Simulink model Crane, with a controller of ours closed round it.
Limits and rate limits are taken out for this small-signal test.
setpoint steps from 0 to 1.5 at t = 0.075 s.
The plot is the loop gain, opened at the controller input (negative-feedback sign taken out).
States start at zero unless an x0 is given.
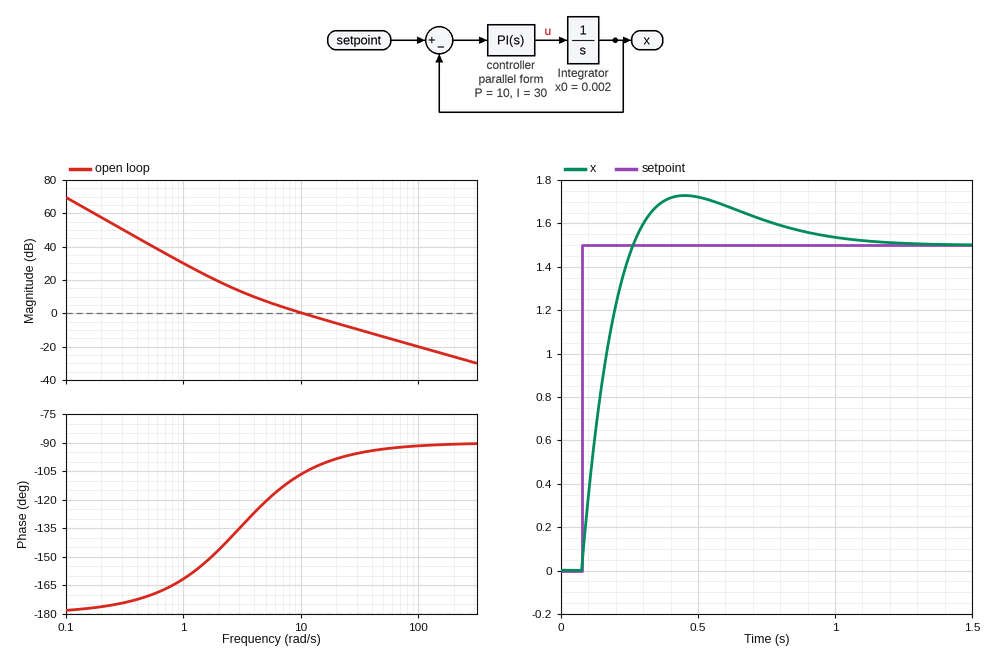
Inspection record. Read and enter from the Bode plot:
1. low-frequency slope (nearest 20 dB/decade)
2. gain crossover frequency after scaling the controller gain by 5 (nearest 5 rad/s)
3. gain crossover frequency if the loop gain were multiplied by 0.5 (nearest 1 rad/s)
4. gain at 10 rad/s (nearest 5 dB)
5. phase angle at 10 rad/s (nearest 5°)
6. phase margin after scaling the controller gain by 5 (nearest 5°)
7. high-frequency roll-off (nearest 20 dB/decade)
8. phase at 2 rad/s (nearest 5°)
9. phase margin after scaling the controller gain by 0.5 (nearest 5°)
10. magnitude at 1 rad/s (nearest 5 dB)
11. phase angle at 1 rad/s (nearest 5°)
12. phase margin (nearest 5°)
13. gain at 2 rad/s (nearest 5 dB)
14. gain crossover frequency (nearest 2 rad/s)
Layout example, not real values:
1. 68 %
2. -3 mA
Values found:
1. -40 dB/decade
2. 50 rad/s
3. 6 rad/s
4. 0 dB
5. -105°
6. 85°
7. -20 dB/decade
8. -145°
9. 60°
10. 30 dB
11. -160°
12. 75°
13. 20 dB
14. 10 rad/s
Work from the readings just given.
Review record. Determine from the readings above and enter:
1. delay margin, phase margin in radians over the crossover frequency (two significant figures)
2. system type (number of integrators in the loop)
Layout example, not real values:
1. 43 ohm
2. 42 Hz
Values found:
1. 0.13 s
2. 2
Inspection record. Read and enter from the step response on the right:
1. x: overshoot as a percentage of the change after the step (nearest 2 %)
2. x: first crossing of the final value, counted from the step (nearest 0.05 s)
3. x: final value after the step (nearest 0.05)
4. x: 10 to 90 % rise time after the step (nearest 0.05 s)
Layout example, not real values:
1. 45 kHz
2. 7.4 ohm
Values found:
1. 16 %
2. 0.20 s
3. 1.50
4. 0.15 s
